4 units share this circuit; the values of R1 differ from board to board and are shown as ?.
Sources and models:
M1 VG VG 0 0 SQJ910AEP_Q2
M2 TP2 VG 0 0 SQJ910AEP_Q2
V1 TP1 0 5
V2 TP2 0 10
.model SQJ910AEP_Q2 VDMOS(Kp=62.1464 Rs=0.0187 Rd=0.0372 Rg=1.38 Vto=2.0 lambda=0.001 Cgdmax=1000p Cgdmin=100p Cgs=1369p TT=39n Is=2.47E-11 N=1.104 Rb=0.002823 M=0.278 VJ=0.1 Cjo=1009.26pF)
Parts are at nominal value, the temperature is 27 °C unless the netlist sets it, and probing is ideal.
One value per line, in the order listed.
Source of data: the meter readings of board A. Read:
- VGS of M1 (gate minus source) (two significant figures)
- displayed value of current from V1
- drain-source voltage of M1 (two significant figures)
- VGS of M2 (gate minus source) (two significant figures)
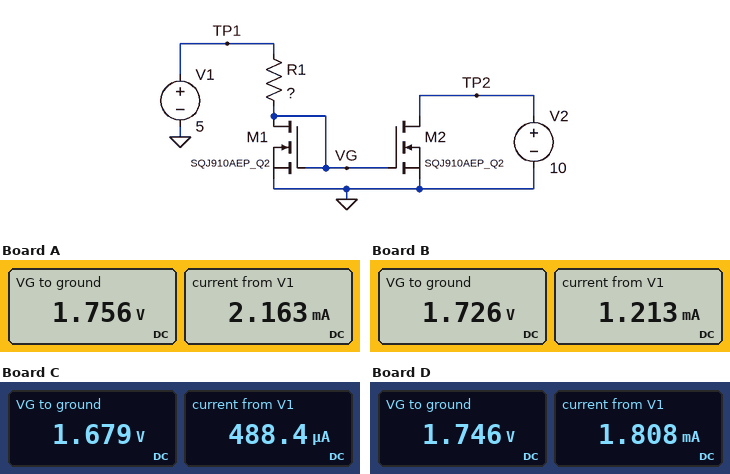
1.8 V
2.163 mA
1.8 V
1.8 V
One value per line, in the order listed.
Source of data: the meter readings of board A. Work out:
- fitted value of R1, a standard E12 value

1.5 kΩ
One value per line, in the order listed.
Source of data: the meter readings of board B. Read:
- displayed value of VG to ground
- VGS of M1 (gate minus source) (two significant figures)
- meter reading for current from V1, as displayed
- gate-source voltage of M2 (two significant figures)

1.726 V
1.7 V
1.213 mA
1.7 V
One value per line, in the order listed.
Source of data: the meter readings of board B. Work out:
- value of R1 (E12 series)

2.7 kΩ
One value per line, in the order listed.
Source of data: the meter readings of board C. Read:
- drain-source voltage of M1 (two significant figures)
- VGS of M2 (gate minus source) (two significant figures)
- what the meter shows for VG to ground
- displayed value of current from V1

1.7 V
1.7 V
1.679 V
488.4 µA
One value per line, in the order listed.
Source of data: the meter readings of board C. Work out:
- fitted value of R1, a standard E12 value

6.8 kΩ
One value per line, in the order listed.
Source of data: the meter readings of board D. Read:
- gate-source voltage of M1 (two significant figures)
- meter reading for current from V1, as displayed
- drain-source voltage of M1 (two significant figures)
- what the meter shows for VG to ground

1.7 V
1.808 mA
1.7 V
1.746 V
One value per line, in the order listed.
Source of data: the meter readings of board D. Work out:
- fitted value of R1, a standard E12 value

1.8 kΩ
